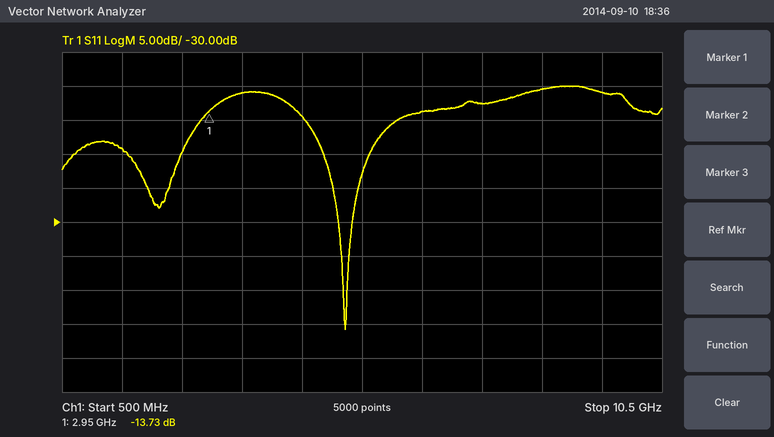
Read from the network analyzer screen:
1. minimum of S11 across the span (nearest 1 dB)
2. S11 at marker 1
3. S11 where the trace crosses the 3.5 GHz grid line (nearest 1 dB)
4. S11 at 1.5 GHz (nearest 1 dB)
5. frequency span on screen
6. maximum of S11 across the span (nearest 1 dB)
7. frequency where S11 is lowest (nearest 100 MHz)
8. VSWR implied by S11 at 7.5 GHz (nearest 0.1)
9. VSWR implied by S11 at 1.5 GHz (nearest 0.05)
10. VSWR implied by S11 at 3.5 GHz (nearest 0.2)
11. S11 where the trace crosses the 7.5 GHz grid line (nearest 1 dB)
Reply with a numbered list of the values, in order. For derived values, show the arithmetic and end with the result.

1. -46 dB
2. -13.73 dB
3. -11 dB
4. -19 dB
5. 10 GHz
6. -10 dB
7. 5.2 GHz
8. |Γ| = 10^(-13/20) = 0.2239; VSWR = (1 + 0.2239)/(1 − 0.2239) ≈ 1.6
9. |Γ| = 10^(-19/20) = 0.1122; VSWR = (1 + 0.1122)/(1 − 0.1122) ≈ 1.25
10. |Γ| = 10^(-11/20) = 0.2818; VSWR = (1 + 0.2818)/(1 − 0.2818) ≈ 1.8
11. -13 dB
